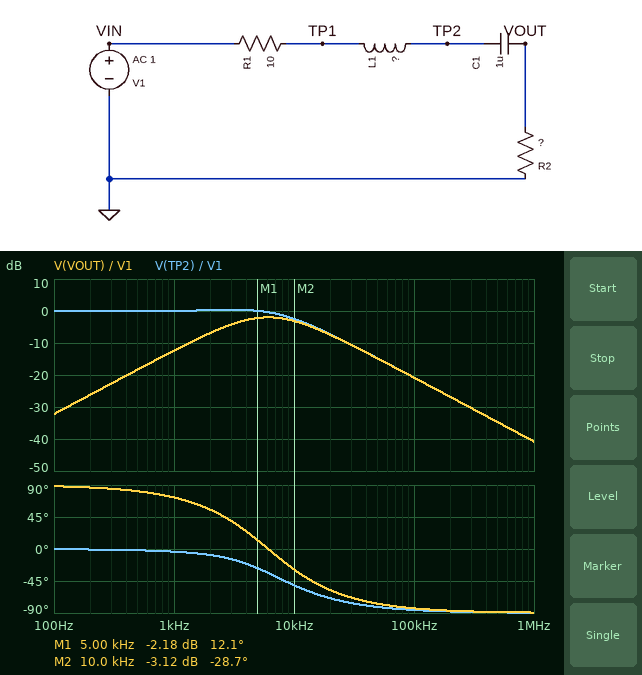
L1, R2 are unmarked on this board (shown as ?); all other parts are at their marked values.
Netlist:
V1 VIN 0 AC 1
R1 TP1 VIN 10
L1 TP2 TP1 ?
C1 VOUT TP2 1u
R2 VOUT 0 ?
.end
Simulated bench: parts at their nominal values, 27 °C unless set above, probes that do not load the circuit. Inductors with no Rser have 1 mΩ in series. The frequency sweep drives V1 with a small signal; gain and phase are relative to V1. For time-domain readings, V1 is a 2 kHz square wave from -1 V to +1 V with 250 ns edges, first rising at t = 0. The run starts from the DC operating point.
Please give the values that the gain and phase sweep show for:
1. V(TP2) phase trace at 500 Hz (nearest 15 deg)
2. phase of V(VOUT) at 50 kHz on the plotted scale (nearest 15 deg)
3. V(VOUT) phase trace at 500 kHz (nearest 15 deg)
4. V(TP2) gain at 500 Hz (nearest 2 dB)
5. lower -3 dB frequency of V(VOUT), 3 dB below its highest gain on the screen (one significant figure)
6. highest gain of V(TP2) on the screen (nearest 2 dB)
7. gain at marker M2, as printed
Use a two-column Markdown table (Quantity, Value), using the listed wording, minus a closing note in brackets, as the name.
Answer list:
| Quantity | Value |
|---|---|
| V(TP2) phase trace at 500 Hz | 0 deg |
| phase of V(VOUT) at 50 kHz on the plotted scale | -75 deg |
| V(VOUT) phase trace at 500 kHz | -90 deg |
| V(TP2) gain at 500 Hz | 0 dB |
| lower -3 dB frequency of V(VOUT), 3 dB below its highest gain on the screen | 3 kHz |
| highest gain of V(TP2) on the screen | 0 dB |
| gain at marker M2, as printed | -3.12 dB |
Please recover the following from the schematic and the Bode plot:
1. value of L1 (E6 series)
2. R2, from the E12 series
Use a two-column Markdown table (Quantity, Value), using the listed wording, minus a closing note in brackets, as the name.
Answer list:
| Quantity | Value |
|---|---|
| value of L1 | 680 µH |
| R2, from the E12 series | 39 Ω |
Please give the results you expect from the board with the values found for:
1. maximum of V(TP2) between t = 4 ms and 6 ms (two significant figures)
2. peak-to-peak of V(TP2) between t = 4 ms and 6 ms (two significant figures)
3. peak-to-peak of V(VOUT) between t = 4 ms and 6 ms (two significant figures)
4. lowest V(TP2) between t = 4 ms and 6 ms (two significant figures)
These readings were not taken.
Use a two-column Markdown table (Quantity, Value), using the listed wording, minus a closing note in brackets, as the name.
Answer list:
| Quantity | Value |
|---|---|
| maximum of V(TP2) between t = 4 ms and 6 ms | 1.1 V |
| peak-to-peak of V(TP2) between t = 4 ms and 6 ms | 2.2 V |
| peak-to-peak of V(VOUT) between t = 4 ms and 6 ms | 2.3 V |
| lowest V(TP2) between t = 4 ms and 6 ms | -1.1 V |
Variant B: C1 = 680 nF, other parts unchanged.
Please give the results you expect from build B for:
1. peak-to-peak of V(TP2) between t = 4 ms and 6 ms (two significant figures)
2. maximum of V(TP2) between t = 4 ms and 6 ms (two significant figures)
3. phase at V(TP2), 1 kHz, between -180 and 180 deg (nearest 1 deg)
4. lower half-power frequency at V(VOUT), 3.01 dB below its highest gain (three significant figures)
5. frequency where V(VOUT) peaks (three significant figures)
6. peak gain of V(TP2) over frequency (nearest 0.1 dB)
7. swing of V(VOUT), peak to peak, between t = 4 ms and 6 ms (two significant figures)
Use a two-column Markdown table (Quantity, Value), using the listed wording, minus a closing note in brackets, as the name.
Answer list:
| Quantity | Value |
|---|---|
| peak-to-peak of V(TP2) between t = 4 ms and 6 ms | 2.4 V |
| maximum of V(TP2) between t = 4 ms and 6 ms | 1.2 V |
| phase at V(TP2), 1 kHz, between -180 and 180 deg | -3 deg |
| lower half-power frequency at V(VOUT), 3.01 dB below its highest gain | 3.63 kHz |
| frequency where V(VOUT) peaks | 7.40 kHz |
| peak gain of V(TP2) over frequency | 0.9 dB |
| swing of V(VOUT), peak to peak, between t = 4 ms and 6 ms | 2.1 V |
